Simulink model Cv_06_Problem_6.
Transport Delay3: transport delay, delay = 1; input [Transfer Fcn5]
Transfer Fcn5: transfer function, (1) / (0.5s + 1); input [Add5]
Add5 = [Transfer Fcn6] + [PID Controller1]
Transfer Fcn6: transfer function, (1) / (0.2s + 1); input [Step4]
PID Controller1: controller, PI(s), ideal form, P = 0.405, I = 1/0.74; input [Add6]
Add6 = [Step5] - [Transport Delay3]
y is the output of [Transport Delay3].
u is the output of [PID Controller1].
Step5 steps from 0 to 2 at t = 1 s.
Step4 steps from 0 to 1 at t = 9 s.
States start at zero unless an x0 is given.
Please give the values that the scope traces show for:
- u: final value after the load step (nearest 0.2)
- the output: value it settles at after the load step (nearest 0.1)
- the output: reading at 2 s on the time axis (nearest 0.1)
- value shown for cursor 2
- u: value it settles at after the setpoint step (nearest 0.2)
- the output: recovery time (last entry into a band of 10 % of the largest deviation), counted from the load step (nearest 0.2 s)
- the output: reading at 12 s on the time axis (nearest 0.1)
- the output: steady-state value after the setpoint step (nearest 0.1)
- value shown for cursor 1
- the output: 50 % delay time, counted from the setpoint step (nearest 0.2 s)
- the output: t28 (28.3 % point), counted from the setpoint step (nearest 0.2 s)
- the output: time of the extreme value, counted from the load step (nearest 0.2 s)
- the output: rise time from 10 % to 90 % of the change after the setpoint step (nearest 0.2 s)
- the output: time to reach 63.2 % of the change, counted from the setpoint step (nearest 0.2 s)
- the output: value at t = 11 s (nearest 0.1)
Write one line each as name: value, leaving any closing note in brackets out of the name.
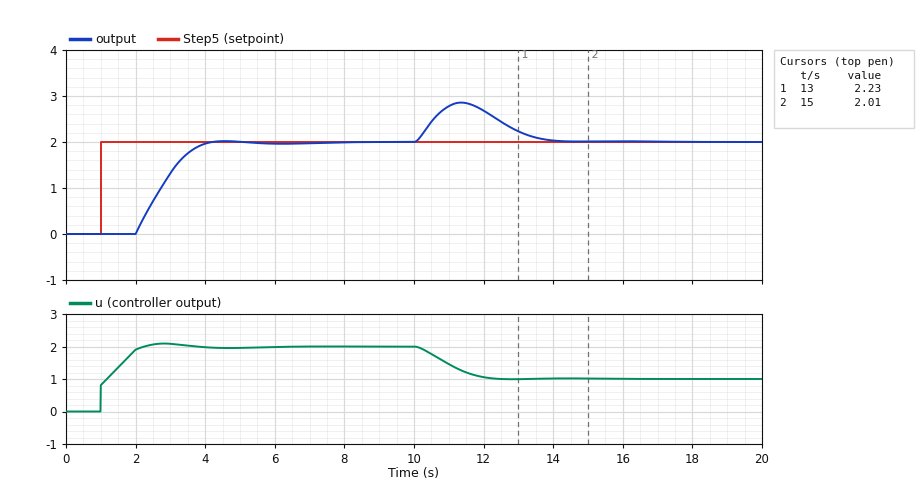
u: final value after the load step: 1.0
the output: value it settles at after the load step: 2.0
the output: reading at 2 s on the time axis: 0.0
value shown for cursor 2: 2.01
u: value it settles at after the setpoint step: 2.0
the output: recovery time (last entry into a band of 10 % of the largest deviation), counted from the load step: 4.6 s
the output: reading at 12 s on the time axis: 2.7
the output: steady-state value after the setpoint step: 2.0
value shown for cursor 1: 2.23
the output: 50 % delay time, counted from the setpoint step: 1.8 s
the output: t28 (28.3 % point), counted from the setpoint step: 1.4 s
the output: time of the extreme value, counted from the load step: 2.4 s
the output: rise time from 10 % to 90 % of the change after the setpoint step: 1.4 s
the output: time to reach 63.2 % of the change, counted from the setpoint step: 2.0 s
the output: value at t = 11 s: 2.8
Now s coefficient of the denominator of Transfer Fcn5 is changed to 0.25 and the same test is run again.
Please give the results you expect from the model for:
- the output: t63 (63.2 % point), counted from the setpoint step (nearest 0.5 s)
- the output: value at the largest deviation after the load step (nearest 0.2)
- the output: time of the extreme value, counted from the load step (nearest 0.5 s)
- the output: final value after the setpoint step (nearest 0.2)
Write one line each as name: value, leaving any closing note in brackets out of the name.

the output: t63 (63.2 % point), counted from the setpoint step: 1.5 s
the output: value at the largest deviation after the load step: 3.0
the output: time of the extreme value, counted from the load step: 2.0 s
the output: final value after the setpoint step: 2.0
